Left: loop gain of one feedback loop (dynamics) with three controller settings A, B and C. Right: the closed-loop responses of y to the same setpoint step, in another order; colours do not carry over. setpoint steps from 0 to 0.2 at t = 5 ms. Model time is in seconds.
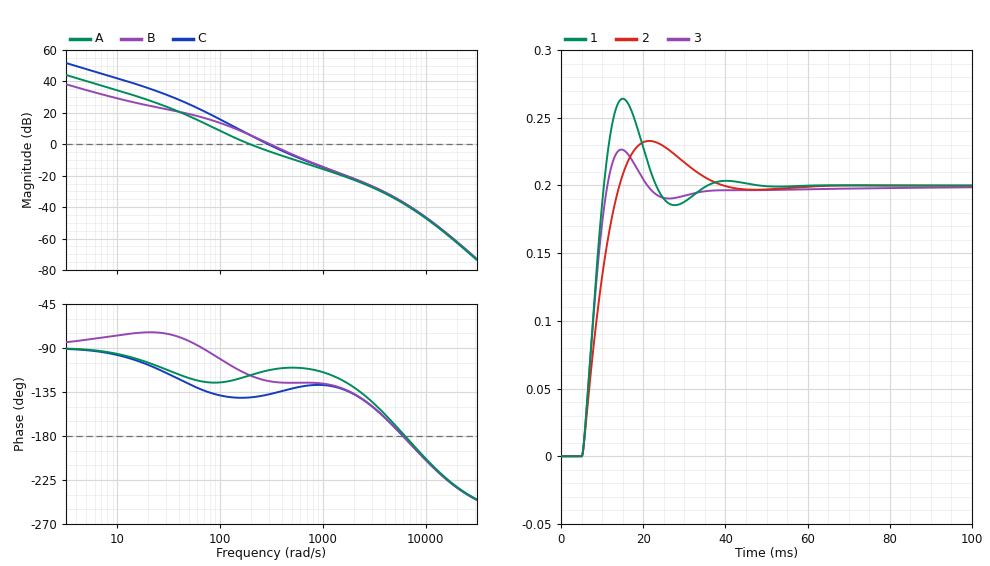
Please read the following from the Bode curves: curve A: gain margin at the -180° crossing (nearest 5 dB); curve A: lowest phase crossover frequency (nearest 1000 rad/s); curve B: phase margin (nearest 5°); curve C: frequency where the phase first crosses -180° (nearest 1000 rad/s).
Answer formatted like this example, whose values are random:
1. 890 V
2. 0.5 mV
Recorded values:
1. 40 dB
2. 6000 rad/s
3. 55°
4. 6000 rad/s
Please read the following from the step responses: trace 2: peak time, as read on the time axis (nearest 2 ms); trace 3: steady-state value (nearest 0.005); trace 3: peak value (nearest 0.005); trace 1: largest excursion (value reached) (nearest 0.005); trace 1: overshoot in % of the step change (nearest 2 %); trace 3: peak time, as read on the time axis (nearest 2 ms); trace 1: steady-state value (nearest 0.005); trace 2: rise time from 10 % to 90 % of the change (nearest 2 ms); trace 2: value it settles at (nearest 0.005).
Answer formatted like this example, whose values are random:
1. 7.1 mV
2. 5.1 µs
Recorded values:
1. 22 ms
2. 0.200
3. 0.225
4. 0.265
5. 32 %
6. 14 ms
7. 0.200
8. 6 ms
9. 0.200
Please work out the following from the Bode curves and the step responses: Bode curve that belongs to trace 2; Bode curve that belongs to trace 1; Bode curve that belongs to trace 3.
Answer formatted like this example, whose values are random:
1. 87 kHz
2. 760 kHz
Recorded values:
1. A
2. C
3. B
